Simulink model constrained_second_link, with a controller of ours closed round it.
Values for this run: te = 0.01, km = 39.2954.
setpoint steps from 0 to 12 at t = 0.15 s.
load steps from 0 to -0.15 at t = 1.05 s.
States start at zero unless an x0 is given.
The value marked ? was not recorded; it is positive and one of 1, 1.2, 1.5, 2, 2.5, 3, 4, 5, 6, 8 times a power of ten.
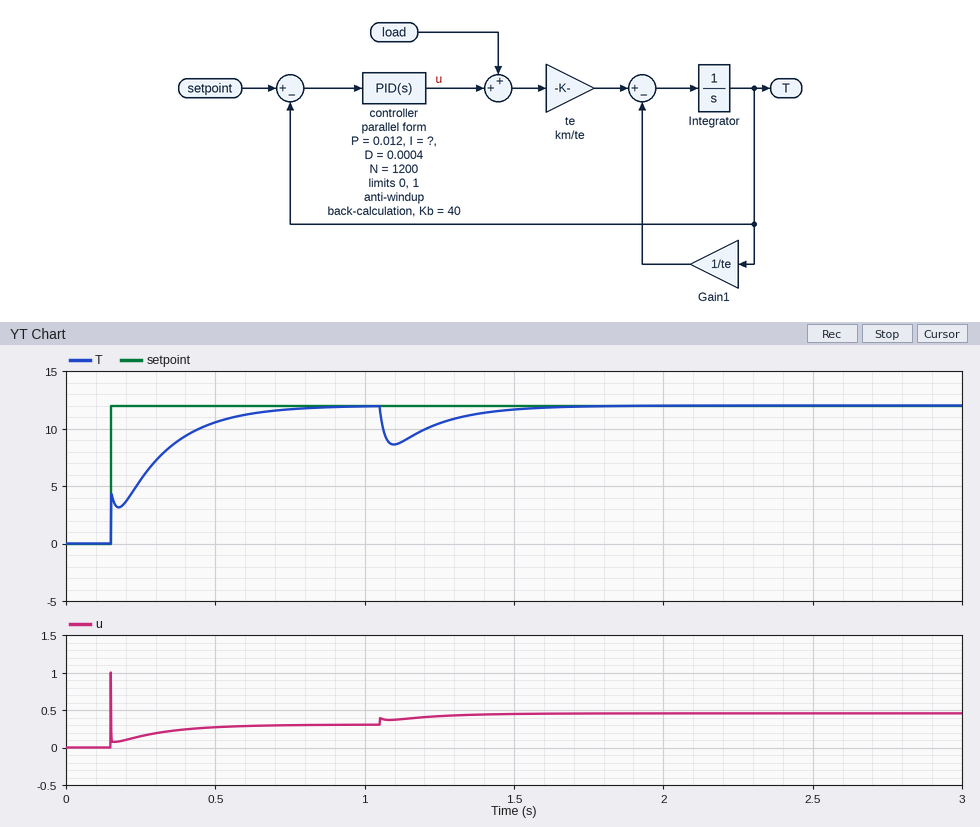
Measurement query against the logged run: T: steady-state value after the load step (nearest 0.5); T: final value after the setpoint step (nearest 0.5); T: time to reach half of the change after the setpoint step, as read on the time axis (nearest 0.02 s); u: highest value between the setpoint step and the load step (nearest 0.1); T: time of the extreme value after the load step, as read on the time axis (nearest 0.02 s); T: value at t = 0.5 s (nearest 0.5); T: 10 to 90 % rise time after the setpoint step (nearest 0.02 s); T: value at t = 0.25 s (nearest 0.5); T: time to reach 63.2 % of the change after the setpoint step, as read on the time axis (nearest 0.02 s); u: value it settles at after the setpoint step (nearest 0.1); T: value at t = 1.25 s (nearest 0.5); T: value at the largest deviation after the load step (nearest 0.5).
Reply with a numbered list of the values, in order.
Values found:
1. 12.0
2. 12.0
3. 0.26 s
4. 1.0
5. 1.10 s
6. 10.5
7. 0.38 s
8. 5.5
9. 0.32 s
10. 0.3
11. 10.5
12. 8.5
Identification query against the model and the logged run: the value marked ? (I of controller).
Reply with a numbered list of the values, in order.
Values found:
1. 0.2
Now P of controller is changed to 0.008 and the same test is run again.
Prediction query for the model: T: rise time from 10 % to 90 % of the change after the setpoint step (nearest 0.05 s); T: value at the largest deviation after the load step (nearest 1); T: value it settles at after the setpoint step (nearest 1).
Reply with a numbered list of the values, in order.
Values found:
1. 0.35 s
2. 8
3. 12
